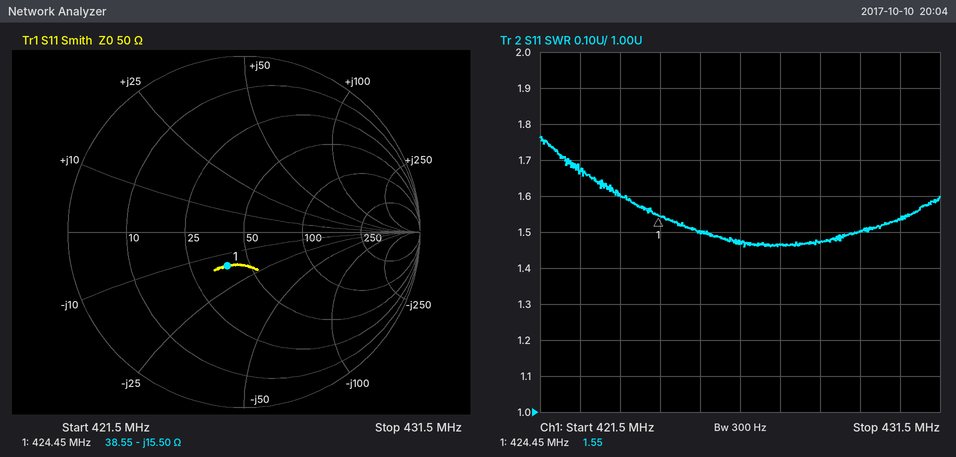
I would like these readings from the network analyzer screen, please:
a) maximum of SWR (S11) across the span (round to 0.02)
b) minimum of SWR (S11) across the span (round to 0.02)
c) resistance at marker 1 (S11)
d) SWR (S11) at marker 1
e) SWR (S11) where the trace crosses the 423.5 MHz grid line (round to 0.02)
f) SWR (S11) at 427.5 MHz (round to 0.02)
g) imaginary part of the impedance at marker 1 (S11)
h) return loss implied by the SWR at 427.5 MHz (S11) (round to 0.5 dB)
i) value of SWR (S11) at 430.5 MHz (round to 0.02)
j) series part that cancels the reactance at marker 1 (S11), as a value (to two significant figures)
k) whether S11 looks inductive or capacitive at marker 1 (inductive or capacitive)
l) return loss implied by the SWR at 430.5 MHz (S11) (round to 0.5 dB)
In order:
1.76
1.46
38.55 Ω
1.55
1.60
1.46
-15.50 Ω
14.5 dB
1.54
5.8 nH
capacitive
13.5 dB
